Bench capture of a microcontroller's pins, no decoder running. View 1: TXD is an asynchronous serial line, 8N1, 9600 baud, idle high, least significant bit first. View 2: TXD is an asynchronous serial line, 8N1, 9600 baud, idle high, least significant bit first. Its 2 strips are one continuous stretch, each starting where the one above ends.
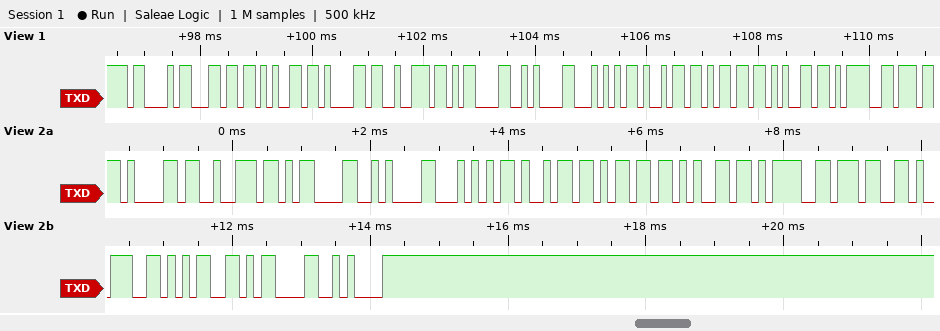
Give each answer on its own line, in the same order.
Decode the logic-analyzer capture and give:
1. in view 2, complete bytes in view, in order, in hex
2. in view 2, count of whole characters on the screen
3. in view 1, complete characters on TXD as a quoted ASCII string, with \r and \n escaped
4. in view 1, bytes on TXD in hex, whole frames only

61 72 0D 0A 54 69 6D 65 3D 37 39 35 0D 0A
14
"Clear\r\nTime="
43 6C 65 61 72 0D 0A 54 69 6D 65 3D
